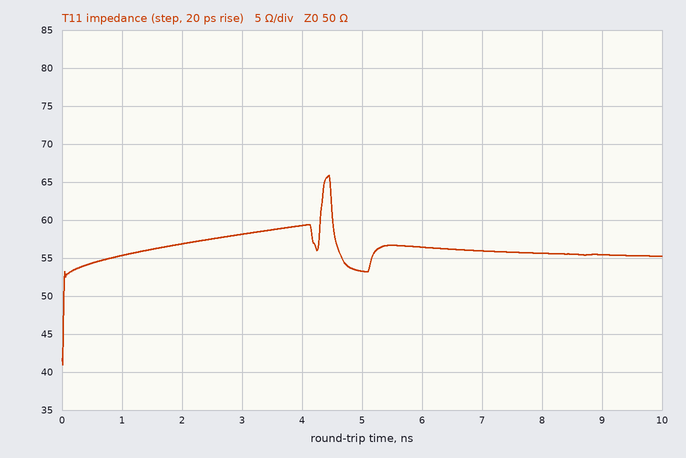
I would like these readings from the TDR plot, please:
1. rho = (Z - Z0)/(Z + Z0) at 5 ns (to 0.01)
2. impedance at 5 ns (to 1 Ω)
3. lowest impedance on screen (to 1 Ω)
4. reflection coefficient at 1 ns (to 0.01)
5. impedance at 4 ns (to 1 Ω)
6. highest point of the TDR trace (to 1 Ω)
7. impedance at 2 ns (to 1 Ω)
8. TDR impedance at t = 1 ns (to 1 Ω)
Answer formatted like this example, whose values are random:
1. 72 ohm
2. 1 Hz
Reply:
1. +0.03
2. 53 Ω
3. 41 Ω
4. +0.05
5. 59 Ω
6. 66 Ω
7. 57 Ω
8. 55 Ω
